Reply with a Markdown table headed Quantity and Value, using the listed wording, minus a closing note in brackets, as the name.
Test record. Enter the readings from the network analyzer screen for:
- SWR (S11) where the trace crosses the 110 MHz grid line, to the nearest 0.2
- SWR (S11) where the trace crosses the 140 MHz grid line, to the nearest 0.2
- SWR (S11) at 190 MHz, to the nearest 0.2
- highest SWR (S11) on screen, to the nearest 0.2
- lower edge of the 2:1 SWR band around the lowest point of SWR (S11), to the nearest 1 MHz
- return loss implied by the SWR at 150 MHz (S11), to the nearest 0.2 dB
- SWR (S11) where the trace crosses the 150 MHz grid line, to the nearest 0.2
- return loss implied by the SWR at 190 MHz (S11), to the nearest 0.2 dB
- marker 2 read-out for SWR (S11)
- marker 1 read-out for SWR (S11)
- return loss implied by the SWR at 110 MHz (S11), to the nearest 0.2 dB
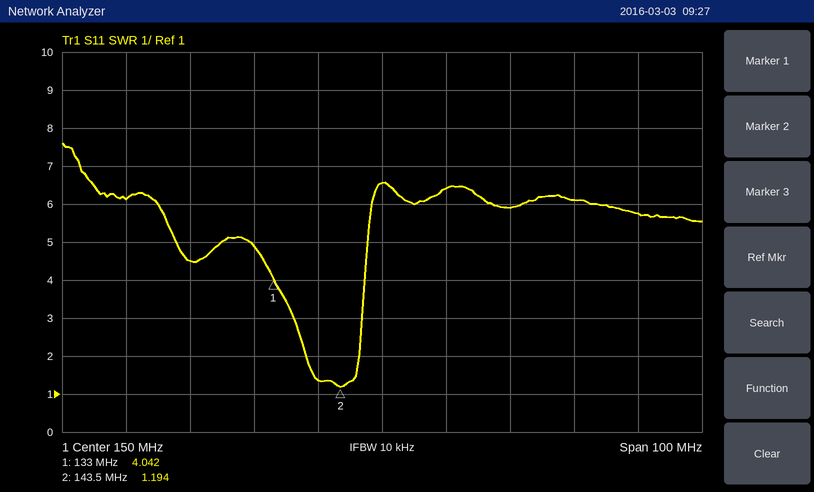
| Quantity | Value |
|---|---|
| SWR (S11) where the trace crosses the 110 MHz grid line, to the nearest 0.2 | 6.2 |
| SWR (S11) where the trace crosses the 140 MHz grid line, to the nearest 0.2 | 1.4 |
| SWR (S11) at 190 MHz, to the nearest 0.2 | 5.8 |
| highest SWR (S11) on screen, to the nearest 0.2 | 7.6 |
| lower edge of the 2:1 SWR band around the lowest point of SWR (S11), to the nearest 1 MHz | 138 MHz |
| return loss implied by the SWR at 150 MHz (S11), to the nearest 0.2 dB | 2.6 dB |
| SWR (S11) where the trace crosses the 150 MHz grid line, to the nearest 0.2 | 6.6 |
| return loss implied by the SWR at 190 MHz (S11), to the nearest 0.2 dB | 3.0 dB |
| marker 2 read-out for SWR | 1.194 |
| marker 1 read-out for SWR | 4.042 |
| return loss implied by the SWR at 110 MHz (S11), to the nearest 0.2 dB | 2.8 dB |
